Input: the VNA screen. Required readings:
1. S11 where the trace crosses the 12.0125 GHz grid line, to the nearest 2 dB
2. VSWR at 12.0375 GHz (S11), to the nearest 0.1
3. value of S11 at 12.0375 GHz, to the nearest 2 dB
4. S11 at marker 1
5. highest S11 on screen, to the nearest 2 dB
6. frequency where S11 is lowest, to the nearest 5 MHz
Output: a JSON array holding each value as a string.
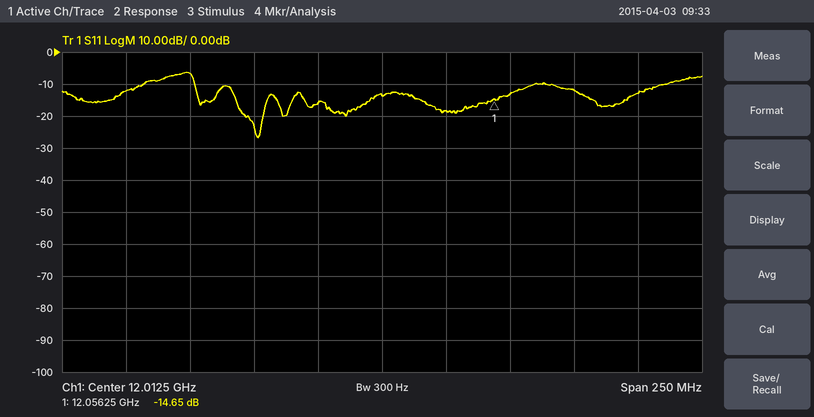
["-14 dB", "1.3", "-18 dB", "-14.65 dB", "-6 dB", "11.965 GHz"]
